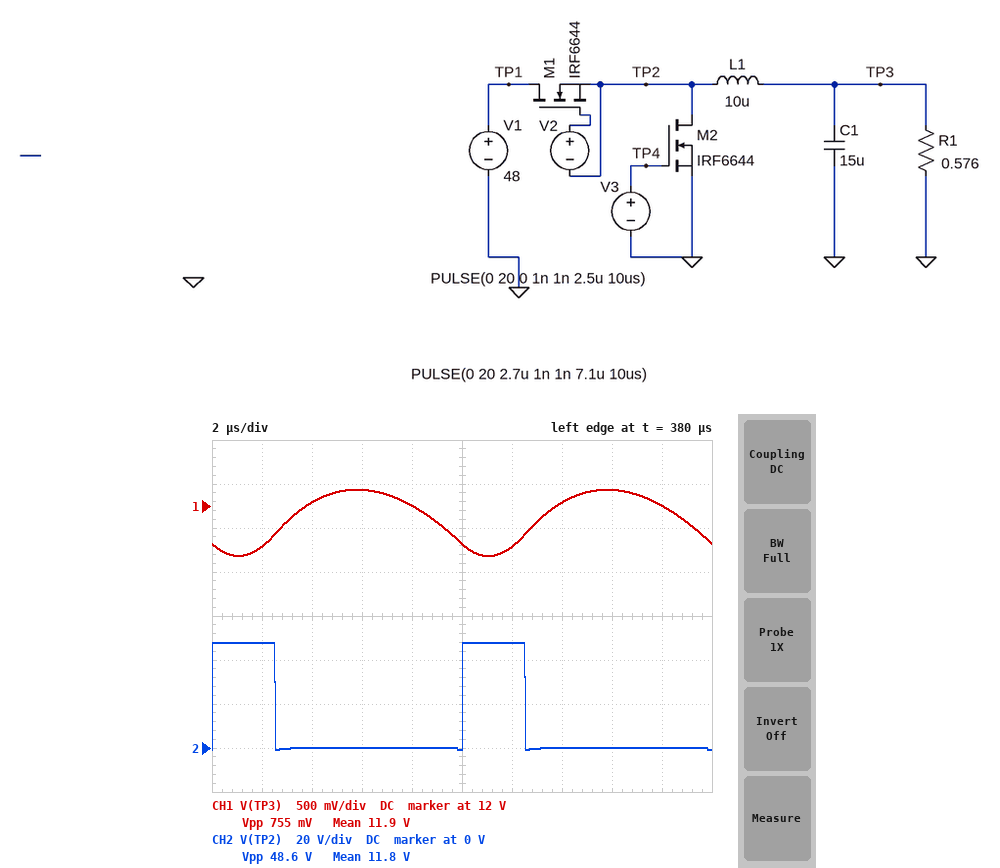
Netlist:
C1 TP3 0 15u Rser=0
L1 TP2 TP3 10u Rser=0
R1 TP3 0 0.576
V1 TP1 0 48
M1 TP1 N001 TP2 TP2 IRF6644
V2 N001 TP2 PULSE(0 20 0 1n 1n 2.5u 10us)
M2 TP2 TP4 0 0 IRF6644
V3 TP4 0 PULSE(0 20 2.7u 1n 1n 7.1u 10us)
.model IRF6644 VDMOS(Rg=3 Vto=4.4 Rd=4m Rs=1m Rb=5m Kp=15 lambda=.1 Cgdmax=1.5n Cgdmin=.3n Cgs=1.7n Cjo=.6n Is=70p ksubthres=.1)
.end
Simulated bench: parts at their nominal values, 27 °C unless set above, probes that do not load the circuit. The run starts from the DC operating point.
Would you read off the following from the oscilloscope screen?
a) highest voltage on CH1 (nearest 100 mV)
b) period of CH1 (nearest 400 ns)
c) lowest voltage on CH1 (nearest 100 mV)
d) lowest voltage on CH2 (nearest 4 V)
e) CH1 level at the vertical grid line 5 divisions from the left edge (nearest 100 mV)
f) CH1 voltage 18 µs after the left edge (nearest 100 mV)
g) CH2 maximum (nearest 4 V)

12.2 V
10.0 µs
11.4 V
0 V
11.6 V
12.0 V
48 V
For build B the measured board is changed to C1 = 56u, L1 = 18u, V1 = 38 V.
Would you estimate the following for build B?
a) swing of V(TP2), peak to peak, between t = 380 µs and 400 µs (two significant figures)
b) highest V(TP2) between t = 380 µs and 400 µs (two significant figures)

39 V
38 V
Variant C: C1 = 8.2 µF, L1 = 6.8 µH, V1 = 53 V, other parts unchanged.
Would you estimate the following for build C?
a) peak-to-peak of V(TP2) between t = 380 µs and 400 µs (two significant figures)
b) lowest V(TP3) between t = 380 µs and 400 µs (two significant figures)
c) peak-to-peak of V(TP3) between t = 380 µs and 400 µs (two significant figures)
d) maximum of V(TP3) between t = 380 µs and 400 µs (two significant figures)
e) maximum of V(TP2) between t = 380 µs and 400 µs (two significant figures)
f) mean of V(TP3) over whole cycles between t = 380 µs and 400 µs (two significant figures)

54 V
12 V
2.2 V
14 V
53 V
13 V
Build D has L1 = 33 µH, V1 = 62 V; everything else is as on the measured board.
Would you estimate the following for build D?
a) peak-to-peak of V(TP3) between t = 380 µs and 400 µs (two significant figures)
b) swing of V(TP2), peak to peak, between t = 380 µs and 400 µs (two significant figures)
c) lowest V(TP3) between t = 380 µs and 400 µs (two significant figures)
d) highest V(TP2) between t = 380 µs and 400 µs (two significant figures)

290 mV
63 V
15 V
62 V
